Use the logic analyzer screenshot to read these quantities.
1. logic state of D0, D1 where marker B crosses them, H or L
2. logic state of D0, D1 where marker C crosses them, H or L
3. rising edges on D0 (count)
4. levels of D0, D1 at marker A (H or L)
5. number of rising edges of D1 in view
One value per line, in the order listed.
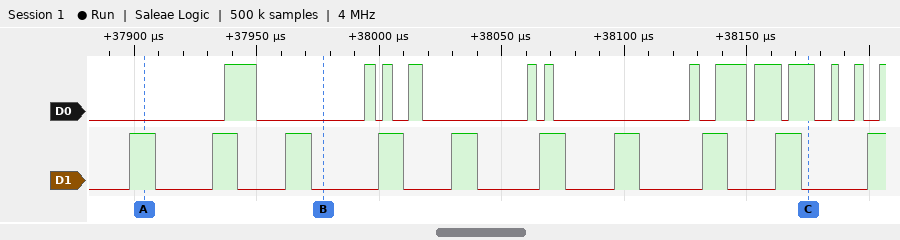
D0=L, D1=L
D0=H, D1=L
13
D0=L, D1=H
10
